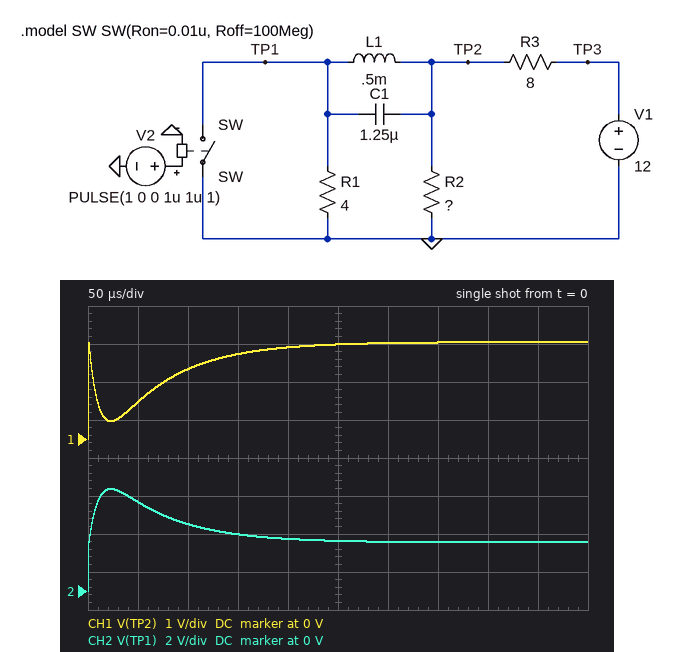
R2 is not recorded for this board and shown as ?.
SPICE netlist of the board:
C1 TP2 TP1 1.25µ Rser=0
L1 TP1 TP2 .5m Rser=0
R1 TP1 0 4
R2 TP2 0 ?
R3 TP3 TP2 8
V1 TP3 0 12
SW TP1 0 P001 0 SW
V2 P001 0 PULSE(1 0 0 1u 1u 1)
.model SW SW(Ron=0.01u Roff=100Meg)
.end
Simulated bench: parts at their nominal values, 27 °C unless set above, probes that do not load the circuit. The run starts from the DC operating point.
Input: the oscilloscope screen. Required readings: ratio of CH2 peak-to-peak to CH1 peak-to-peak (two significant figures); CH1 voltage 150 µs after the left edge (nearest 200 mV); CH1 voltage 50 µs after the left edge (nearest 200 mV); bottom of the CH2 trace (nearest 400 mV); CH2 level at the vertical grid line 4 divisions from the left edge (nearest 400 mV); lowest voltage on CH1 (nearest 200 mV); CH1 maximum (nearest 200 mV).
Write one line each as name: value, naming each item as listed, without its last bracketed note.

ratio of CH2 peak-to-peak to CH1 peak-to-peak: 2.1
CH1 voltage 150 µs after the left edge: 2.2 V
CH1 voltage 50 µs after the left edge: 1.0 V
bottom of the CH2 trace: 0 V
CH2 level at the vertical grid line 4 divisions from the left edge: 2.8 V
lowest voltage on CH1: 0 V
CH1 maximum: 2.6 V
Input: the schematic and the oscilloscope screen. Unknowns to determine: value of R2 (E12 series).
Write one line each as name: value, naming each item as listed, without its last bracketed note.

value of R2: 4.7 Ω
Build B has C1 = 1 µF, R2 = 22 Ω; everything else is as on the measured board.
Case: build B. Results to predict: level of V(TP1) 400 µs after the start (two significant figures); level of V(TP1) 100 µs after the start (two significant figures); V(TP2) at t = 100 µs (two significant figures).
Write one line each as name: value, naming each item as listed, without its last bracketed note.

level of V(TP1) 400 µs after the start: 3.6 V
level of V(TP1) 100 µs after the start: 3.9 V
V(TP2) at t = 100 µs: 3.0 V
